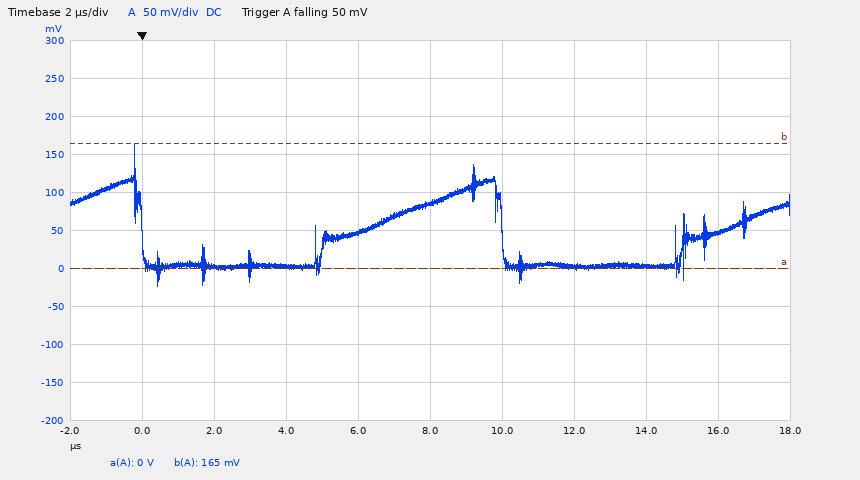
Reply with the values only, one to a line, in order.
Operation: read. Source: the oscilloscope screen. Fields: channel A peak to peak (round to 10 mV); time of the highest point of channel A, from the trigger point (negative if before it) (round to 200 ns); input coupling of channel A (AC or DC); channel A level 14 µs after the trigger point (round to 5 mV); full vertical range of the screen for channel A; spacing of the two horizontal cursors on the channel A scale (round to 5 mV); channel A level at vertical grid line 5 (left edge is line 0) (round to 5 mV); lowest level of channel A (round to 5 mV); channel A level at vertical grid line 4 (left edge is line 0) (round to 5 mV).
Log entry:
190 mV
-200 ns
DC
5 mV
500 mV
165 mV
85 mV
-25 mV
45 mV
